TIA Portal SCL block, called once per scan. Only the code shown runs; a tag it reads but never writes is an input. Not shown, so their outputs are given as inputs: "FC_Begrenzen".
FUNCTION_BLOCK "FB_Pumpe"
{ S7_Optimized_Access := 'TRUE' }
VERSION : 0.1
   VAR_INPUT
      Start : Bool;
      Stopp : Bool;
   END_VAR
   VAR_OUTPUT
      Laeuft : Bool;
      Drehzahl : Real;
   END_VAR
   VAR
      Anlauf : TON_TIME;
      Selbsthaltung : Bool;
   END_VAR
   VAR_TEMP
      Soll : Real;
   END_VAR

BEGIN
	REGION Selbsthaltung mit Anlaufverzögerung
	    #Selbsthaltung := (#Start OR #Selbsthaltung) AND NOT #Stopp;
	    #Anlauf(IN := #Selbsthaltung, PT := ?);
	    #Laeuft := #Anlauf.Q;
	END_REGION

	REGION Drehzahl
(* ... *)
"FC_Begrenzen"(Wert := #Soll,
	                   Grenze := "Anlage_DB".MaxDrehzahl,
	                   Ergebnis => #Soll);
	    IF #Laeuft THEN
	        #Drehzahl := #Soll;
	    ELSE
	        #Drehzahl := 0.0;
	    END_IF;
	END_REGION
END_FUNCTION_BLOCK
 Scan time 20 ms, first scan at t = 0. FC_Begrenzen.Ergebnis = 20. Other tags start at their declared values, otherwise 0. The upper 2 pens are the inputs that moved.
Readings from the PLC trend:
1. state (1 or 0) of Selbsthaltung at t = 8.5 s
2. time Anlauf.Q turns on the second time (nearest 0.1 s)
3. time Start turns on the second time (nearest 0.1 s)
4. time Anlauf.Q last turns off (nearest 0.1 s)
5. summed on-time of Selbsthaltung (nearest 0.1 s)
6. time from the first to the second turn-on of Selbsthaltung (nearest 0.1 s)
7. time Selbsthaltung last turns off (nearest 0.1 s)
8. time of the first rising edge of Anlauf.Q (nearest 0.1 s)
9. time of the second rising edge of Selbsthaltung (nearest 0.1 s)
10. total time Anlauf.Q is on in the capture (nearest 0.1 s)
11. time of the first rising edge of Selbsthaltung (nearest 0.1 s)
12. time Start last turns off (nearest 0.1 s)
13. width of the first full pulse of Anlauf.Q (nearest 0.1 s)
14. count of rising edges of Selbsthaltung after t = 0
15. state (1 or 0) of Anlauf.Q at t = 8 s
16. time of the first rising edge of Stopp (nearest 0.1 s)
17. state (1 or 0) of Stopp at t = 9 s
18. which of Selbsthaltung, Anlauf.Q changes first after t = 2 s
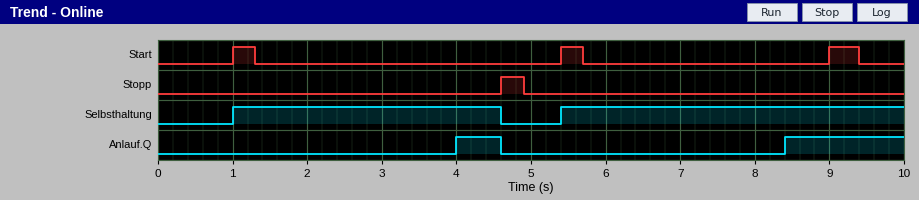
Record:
1
8.4 s
5.4 s
4.6 s
8.2 s
4.4 s
4.6 s
4.0 s
5.4 s
2.2 s
1.0 s
9.4 s
0.6 s
2
0
4.6 s
0
Anlauf.Q
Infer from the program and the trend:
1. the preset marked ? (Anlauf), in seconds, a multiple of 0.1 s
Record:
3.0 s
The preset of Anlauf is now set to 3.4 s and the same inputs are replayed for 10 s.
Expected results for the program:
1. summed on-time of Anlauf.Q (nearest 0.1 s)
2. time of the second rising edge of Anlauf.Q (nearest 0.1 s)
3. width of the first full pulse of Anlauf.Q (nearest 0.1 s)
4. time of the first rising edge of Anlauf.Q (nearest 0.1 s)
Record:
1.4 s
8.8 s
0.2 s
4.4 s
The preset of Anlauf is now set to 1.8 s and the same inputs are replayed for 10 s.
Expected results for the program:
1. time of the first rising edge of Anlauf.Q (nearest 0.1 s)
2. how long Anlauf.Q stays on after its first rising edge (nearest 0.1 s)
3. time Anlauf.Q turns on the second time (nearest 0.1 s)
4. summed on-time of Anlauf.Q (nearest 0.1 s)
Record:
2.8 s
1.8 s
7.2 s
4.6 s
